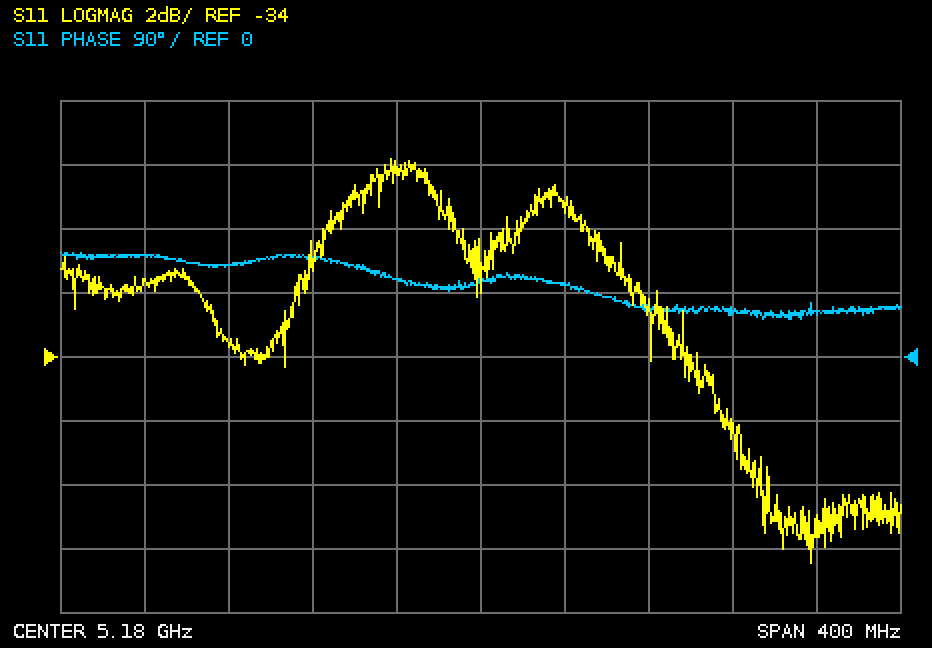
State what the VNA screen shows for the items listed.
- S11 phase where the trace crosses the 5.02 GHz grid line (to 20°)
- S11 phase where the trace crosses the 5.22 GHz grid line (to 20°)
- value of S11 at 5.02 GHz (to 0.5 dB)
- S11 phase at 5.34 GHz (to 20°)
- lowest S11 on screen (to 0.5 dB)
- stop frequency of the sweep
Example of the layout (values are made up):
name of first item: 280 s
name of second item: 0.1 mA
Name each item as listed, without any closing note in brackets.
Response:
S11 phase where the trace crosses the 5.02 GHz grid line: 140°
S11 phase where the trace crosses the 5.22 GHz grid line: 100°
value of S11 at 5.02 GHz: -31.5 dB
S11 phase at 5.34 GHz: 60°
lowest S11 on screen: -40.5 dB
stop frequency of the sweep: 5.38 GHz
